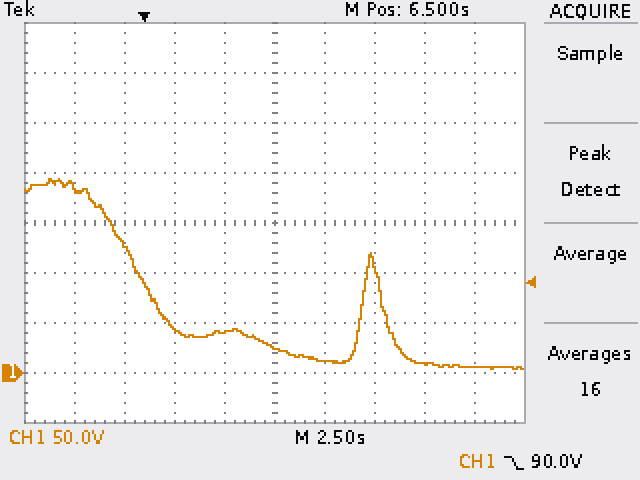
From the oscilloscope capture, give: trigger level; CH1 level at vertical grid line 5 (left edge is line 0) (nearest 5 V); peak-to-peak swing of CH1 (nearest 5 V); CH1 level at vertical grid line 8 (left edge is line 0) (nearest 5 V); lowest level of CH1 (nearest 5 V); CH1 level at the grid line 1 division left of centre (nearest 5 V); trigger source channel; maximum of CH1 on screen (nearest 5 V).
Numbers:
90.0 V
25 V
190 V
10 V
5 V
40 V
CH1
195 V
